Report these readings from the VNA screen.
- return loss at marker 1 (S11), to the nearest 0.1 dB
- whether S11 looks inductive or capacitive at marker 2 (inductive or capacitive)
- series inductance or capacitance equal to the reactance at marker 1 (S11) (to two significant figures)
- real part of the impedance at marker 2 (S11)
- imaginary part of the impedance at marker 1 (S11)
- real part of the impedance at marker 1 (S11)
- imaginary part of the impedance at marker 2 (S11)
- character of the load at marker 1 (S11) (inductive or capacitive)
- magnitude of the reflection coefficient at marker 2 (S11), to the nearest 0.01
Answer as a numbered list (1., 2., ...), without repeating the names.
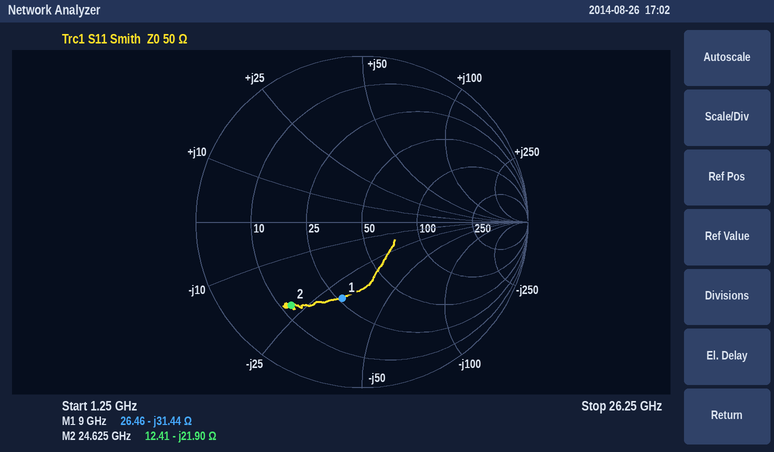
1. 6.5 dB
2. capacitive
3. 560 fF
4. 12.41 Ω
5. -31.44 Ω
6. 26.46 Ω
7. -21.90 Ω
8. capacitive
9. 0.66
